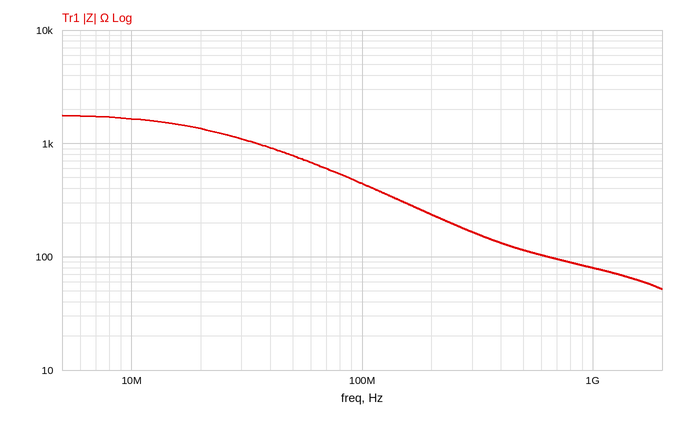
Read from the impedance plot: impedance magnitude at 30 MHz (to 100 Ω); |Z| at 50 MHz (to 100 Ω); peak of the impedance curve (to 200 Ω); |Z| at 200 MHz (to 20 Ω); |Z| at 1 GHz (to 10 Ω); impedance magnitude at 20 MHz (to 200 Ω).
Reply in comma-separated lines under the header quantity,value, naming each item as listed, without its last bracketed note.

quantity,value
impedance magnitude at 30 MHz,1.1 kΩ
|Z| at 50 MHz,800 Ω
peak of the impedance curve,1.8 kΩ
|Z| at 200 MHz,240 Ω
|Z| at 1 GHz,80 Ω
impedance magnitude at 20 MHz,1.4 kΩ
